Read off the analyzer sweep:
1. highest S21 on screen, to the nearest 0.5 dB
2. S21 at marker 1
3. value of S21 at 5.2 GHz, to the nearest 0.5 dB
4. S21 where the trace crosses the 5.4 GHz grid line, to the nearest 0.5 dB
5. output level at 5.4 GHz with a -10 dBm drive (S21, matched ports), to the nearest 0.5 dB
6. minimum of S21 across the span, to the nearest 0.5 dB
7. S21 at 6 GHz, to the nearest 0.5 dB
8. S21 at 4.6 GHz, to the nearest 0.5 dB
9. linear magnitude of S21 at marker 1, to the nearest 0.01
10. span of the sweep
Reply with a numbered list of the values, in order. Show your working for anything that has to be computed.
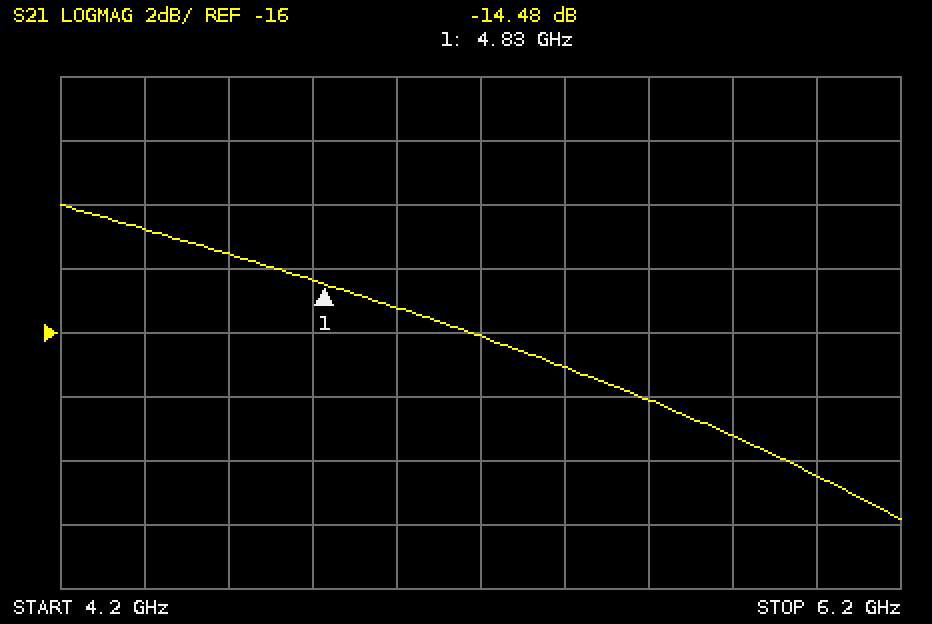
1. -12.0 dB
2. -14.48 dB
3. -16.0 dB
4. -17.0 dB
5. -10 dBm + (-17.0 dB) = -27.0 dBm
6. -22.0 dB
7. -20.5 dB
8. -13.5 dB
9. 10^(-14.48/20) ≈ 0.19
10. 2 GHz
